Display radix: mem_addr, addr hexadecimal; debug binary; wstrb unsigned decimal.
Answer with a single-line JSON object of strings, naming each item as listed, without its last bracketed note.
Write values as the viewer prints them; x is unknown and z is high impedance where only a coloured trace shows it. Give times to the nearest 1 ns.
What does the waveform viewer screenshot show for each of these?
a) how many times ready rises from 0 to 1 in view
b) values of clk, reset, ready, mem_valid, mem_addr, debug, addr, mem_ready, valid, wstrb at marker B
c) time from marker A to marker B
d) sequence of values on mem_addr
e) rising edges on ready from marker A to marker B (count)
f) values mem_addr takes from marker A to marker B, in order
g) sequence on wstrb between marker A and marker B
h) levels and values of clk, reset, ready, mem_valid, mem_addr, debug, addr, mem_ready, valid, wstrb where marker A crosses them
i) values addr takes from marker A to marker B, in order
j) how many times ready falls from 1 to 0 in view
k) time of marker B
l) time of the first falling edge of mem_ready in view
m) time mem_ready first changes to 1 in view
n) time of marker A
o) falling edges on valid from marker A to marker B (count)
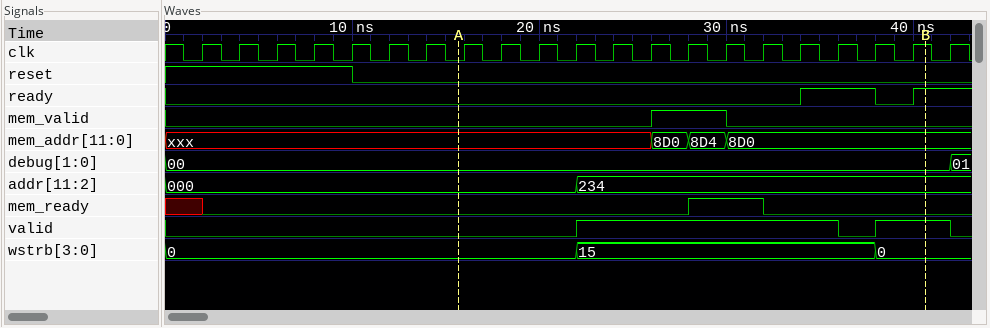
{"how many times ready rises from 0 to 1 in view": "2", "values of clk, reset, ready, mem_valid, mem_addr, debug, addr, mem_ready, valid, wstrb at marker B": "clk=1, reset=0, ready=1, mem_valid=0, mem_addr=8D0, debug=00, addr=234, mem_ready=0, valid=1, wstrb=0", "time from marker A to marker B": "25 ns", "sequence of values on mem_addr": "xxx, 8D0, 8D4, 8D0", "rising edges on ready from marker A to marker B": "2", "values mem_addr takes from marker A to marker B, in order": "xxx, 8D0, 8D4, 8D0", "sequence on wstrb between marker A and marker B": "0, 15, 0", "levels and values of clk, reset, ready, mem_valid, mem_addr, debug, addr, mem_ready, valid, wstrb where marker A crosses them": "clk=0, reset=0, ready=0, mem_valid=0, mem_addr=xxx, debug=00, addr=000, mem_ready=0, valid=0, wstrb=0", "values addr takes from marker A to marker B, in order": "000, 234", "how many times ready falls from 1 to 0 in view": "1", "time of marker B": "41 ns", "time of the first falling edge of mem_ready in view": "32 ns", "time mem_ready first changes to 1 in view": "28 ns", "time of marker A": "16 ns", "falling edges on valid from marker A to marker B": "1"}
